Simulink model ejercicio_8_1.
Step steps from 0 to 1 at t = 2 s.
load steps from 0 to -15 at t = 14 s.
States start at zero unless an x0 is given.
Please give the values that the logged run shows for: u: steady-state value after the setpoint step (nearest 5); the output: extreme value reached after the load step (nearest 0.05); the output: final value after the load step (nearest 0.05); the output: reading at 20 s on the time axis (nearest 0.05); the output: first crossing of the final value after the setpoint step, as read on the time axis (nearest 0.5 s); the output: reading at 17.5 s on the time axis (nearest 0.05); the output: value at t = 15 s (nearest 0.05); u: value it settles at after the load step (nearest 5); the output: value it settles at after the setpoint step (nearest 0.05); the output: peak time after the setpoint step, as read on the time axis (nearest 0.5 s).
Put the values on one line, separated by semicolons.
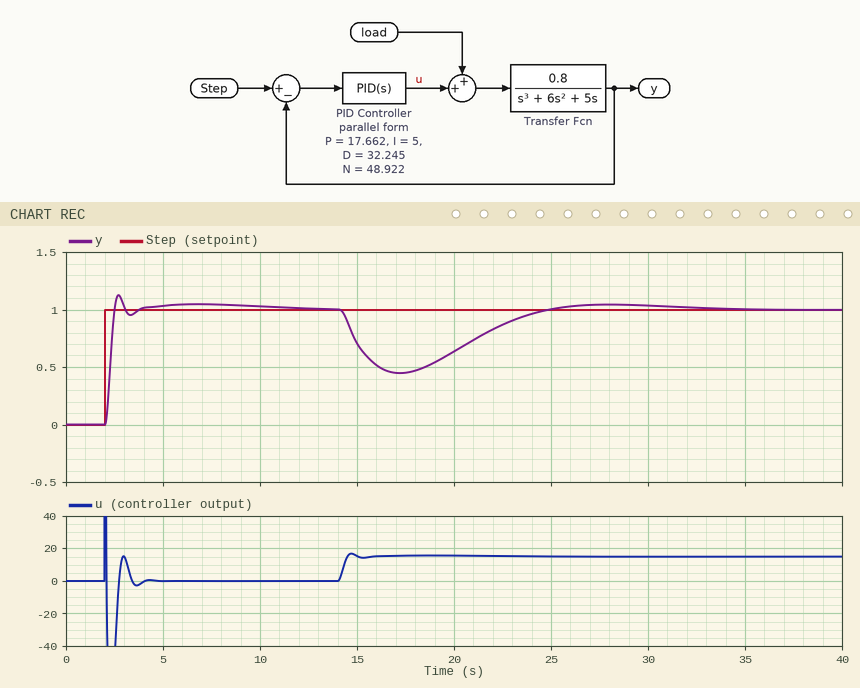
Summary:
0; 0.45; 1.00; 0.65; 2.5 s; 0.45; 0.70; 15; 1.00; 2.5 s
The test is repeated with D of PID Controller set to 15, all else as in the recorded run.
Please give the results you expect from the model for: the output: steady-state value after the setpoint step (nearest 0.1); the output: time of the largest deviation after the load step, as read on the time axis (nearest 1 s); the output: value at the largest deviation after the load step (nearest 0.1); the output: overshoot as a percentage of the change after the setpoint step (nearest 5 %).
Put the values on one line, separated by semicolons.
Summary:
1.0; 16 s; 0.3; 15 %
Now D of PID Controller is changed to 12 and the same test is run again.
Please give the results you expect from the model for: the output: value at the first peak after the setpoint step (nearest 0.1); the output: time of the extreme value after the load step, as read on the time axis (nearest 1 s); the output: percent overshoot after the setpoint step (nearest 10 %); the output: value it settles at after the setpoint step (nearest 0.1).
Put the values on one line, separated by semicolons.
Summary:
1.2; 16 s; 20 %; 1.0
